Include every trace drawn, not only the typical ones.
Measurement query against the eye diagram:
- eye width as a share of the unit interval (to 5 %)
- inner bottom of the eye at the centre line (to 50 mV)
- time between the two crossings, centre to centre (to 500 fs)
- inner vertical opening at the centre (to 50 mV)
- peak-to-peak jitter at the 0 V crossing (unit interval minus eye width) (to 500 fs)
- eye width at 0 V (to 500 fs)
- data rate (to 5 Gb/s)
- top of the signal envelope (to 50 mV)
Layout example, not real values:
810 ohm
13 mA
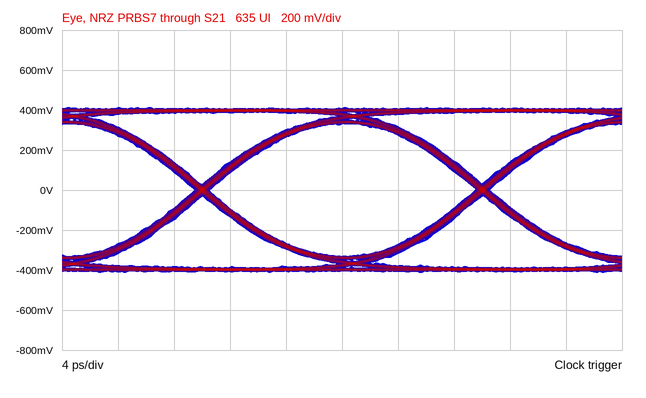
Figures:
95 %
-350 mV
20.0 ps
650 mV
1.0 ps
19.0 ps
50 Gb/s
400 mV
